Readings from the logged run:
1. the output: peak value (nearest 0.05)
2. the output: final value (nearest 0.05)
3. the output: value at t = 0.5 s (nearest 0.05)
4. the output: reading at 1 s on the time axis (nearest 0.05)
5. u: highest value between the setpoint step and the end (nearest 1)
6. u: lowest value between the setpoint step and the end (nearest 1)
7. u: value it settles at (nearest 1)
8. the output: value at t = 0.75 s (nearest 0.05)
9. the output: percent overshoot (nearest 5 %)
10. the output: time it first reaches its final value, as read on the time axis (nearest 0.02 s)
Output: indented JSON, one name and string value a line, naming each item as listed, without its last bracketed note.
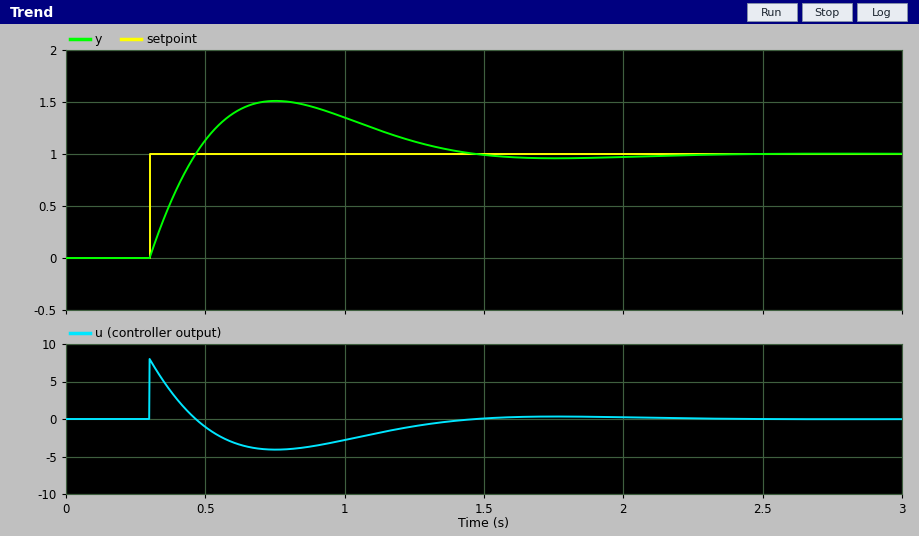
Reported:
{
  "the output: peak value": "1.50",
  "the output: final value": "1.00",
  "the output: value at t = 0.5 s": "1.15",
  "the output: reading at 1 s on the time axis": "1.35",
  "u: highest value between the setpoint step and the end": "8",
  "u: lowest value between the setpoint step and the end": "-4",
  "u: value it settles at": "0",
  "the output: value at t = 0.75 s": "1.50",
  "the output: percent overshoot": "50 %",
  "the output: time it first reaches its final value, as read on the time axis": "0.46 s"
}
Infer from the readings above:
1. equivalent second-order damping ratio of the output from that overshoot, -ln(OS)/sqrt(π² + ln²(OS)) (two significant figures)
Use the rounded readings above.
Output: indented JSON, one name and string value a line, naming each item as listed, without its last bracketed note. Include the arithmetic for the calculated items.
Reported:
{
  "equivalent second-order damping ratio of the output from that overshoot, -ln(OS)/sqrt(π² + ln²(OS))": "ln(0.5) = -0.693; 0.693 / sqrt(9.870 + 0.480) = 0.22"
}
